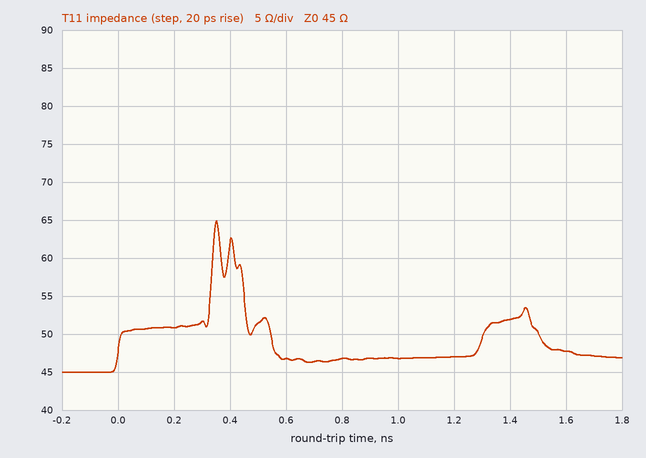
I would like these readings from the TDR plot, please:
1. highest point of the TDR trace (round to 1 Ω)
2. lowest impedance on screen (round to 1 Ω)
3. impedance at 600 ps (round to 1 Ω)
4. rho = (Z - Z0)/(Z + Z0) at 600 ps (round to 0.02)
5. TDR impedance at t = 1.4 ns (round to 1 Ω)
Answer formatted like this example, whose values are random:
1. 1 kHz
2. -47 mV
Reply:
1. 65 Ω
2. 45 Ω
3. 47 Ω
4. +0.02
5. 52 Ω
